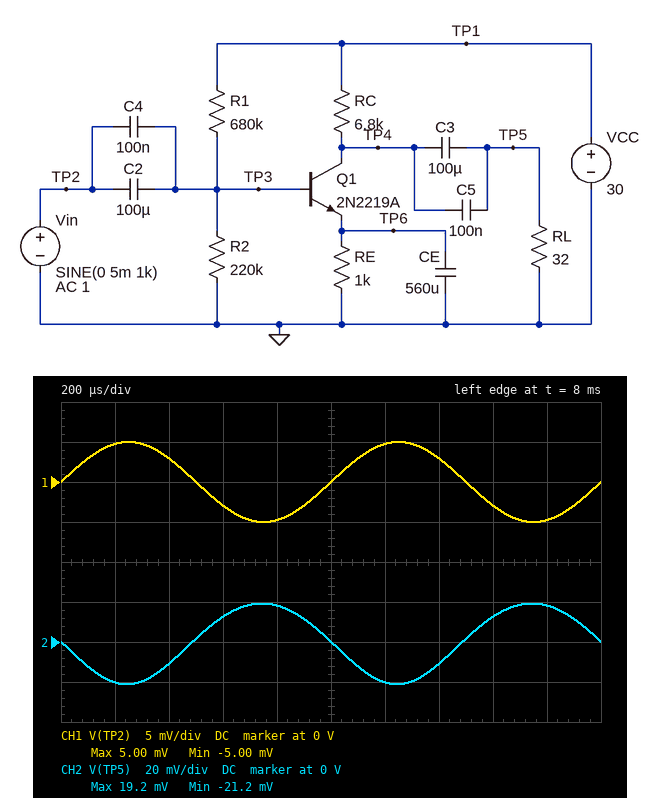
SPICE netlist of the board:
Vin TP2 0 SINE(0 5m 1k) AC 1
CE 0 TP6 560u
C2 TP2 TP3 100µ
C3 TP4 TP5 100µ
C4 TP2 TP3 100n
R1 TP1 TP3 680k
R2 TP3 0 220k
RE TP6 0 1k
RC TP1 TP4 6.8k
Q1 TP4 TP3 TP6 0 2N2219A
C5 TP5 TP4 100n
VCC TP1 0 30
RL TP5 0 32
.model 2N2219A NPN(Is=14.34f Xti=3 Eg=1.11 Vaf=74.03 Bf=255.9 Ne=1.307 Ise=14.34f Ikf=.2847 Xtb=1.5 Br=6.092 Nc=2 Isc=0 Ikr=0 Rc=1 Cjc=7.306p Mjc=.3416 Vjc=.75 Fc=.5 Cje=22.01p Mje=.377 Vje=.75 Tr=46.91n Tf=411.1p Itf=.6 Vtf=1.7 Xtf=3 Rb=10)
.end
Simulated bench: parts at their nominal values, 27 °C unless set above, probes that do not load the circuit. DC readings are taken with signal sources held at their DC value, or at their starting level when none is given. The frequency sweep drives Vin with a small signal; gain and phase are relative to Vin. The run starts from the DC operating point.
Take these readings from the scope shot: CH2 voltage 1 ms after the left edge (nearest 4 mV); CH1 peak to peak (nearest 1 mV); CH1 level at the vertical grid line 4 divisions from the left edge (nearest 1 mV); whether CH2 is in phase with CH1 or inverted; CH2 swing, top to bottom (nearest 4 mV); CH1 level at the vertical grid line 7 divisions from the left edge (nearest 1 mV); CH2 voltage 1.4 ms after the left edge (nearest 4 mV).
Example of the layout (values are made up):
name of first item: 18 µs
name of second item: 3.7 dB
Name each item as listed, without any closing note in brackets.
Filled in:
CH2 voltage 1 ms after the left edge: 0 V
CH1 peak to peak: 10 mV
CH1 level at the vertical grid line 4 divisions from the left edge: -5 mV
whether CH2 is in phase with CH1 or inverted: inverted
CH2 swing, top to bottom: 40 mV
CH1 level at the vertical grid line 7 divisions from the left edge: 3 mV
CH2 voltage 1.4 ms after the left edge: -12 mV
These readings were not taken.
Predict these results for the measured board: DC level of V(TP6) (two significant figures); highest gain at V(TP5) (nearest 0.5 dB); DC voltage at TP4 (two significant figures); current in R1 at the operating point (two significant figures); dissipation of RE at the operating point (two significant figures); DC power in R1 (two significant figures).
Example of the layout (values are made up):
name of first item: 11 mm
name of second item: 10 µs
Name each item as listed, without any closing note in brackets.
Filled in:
DC level of V(TP6): 3.4 V
highest gain at V(TP5): 12.0 dB
DC voltage at TP4: 7.2 V
current in R1 at the operating point: 38 µA
dissipation of RE at the operating point: 11 mW
DC power in R1: 990 µW
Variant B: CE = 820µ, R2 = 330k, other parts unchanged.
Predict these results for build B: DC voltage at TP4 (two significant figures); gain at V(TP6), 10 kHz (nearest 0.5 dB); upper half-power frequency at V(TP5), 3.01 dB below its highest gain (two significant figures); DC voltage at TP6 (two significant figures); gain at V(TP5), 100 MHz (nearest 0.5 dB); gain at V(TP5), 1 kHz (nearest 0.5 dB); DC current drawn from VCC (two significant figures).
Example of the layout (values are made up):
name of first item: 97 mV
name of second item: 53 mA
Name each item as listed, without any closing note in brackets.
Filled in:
DC voltage at TP4: 4.0 V
gain at V(TP6), 10 kHz: -51.0 dB
upper half-power frequency at V(TP5), 3.01 dB below its highest gain: 74 MHz
DC voltage at TP6: 3.8 V
gain at V(TP5), 100 MHz: 8.5 dB
gain at V(TP5), 1 kHz: 13.0 dB
DC current drawn from VCC: 3.9 mA
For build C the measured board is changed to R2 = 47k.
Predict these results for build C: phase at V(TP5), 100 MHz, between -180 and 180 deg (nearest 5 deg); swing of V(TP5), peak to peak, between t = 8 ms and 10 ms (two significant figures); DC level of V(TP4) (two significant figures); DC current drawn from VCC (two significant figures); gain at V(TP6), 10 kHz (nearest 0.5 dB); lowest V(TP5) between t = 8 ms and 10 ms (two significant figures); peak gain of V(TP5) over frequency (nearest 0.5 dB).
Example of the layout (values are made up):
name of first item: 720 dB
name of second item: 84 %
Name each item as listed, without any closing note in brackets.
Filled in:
phase at V(TP5), 100 MHz, between -180 and 180 deg: 155 deg
swing of V(TP5), peak to peak, between t = 8 ms and 10 ms: 13 mV
DC level of V(TP4): 23 V
DC current drawn from VCC: 1.1 mA
gain at V(TP6), 10 kHz: -59.0 dB
lowest V(TP5) between t = 8 ms and 10 ms: -6.8 mV
peak gain of V(TP5) over frequency: 2.0 dB
